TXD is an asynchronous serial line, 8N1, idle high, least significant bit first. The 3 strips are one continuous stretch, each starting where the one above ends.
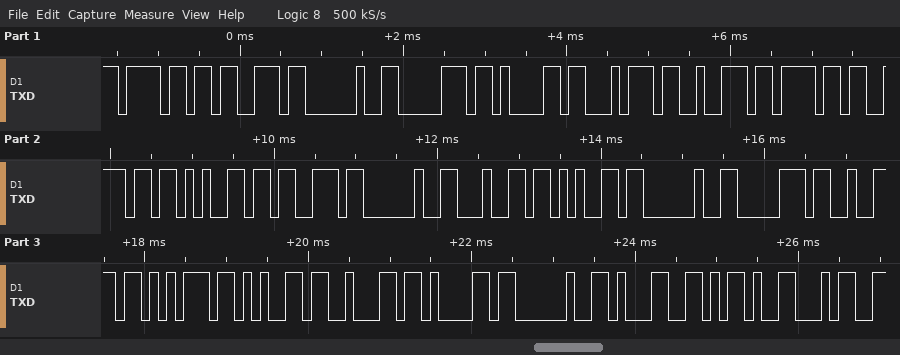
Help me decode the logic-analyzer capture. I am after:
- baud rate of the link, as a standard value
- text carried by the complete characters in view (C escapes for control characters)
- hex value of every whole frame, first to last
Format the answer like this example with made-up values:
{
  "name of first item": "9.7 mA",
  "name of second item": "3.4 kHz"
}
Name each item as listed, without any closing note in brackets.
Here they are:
{
  "baud rate of the link, as a standard value": "9600 baud",
  "text carried by the complete characters in view": "\"os patrones de prueba 1-4\"",
  "hex value of every whole frame, first to last": "0x6F 0x73 0x20 0x70 0x61 0x74 0x72 0x6F 0x6E 0x65 0x73 0x20 0x64 0x65 0x20 0x70 0x72 0x75 0x65 0x62 0x61 0x20 0x31 0x2D 0x34"
}
